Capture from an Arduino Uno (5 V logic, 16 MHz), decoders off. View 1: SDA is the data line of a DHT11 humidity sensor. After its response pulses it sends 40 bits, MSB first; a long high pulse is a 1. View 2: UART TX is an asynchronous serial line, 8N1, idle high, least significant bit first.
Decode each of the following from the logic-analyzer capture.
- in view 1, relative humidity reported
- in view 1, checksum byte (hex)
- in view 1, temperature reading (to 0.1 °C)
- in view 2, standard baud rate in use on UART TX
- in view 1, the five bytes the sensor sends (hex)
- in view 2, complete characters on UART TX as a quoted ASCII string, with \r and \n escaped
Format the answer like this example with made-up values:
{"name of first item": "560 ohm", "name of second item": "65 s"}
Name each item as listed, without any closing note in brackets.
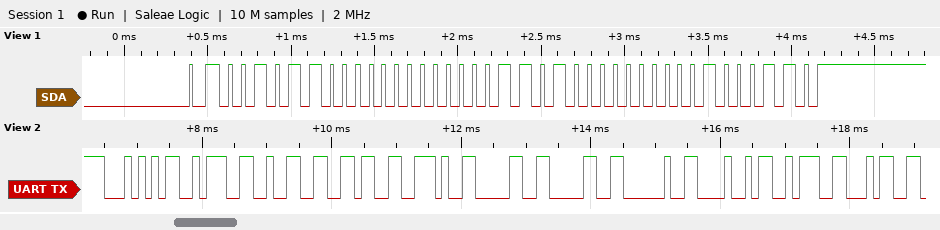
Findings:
{"in view 1, relative humidity reported": "44 %", "in view 1, checksum byte": "0x46", "in view 1, temperature reading": "26.0 °C", "in view 2, standard baud rate in use on UART TX": "9600 baud", "in view 1, the five bytes the sensor sends": "2C 00 1A 00 46", "in view 2, complete characters on UART TX as a quoted ASCII string, with \\r and \\n escaped": "\"T:26.00 H:4\""}
